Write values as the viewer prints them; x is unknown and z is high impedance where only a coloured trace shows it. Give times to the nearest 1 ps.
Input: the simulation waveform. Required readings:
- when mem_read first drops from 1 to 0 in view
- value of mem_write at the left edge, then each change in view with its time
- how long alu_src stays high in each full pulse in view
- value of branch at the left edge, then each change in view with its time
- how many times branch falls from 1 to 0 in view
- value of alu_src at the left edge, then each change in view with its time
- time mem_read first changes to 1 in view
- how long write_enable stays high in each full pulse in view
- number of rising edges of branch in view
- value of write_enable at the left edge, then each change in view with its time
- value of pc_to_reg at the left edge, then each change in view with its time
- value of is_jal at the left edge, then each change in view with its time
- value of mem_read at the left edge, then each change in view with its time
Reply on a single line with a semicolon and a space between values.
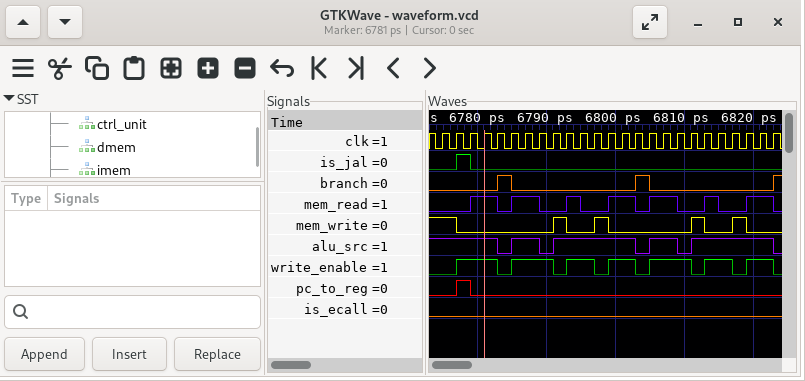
6783 ps; 1, 0 at 6777 ps, 1 at 6791 ps, 0 at 6793 ps, 1 at 6797 ps, 0 at 6799 ps, 1 at 6811 ps, 0 at 6813 ps, 1 at 6817 ps, 0 at 6819 ps; 4 ps, 12 ps, 4 ps, 12 ps; 0, 1 at 6783 ps, 0 at 6785 ps, 1 at 6803 ps, 0 at 6805 ps, 1 at 6823 ps; 2; 1, 0 at 6783 ps, 1 at 6785 ps, 0 at 6789 ps, 1 at 6791 ps, 0 at 6803 ps, 1 at 6805 ps, 0 at 6809 ps, 1 at 6811 ps, 0 at 6823 ps; 6779 ps; 6 ps, 6 ps, 4 ps, 4 ps, 6 ps, 4 ps, 4 ps; 3; 0, 1 at 6777 ps, 0 at 6783 ps, 1 at 6785 ps, 0 at 6791 ps, 1 at 6793 ps, 0 at 6797 ps, 1 at 6799 ps, 0 at 6803 ps, 1 at 6805 ps, 0 at 6811 ps, 1 at 6813 ps, 0 at 6817 ps, 1 at 6819 ps, 0 at 6823 ps; 0, 1 at 6777 ps, 0 at 6779 ps; 0, 1 at 6777 ps, 0 at 6779 ps; 0, 1 at 6779 ps, 0 at 6783 ps, 1 at 6785 ps, 0 at 6789 ps, 1 at 6793 ps, 0 at 6795 ps, 1 at 6799 ps, 0 at 6803 ps, 1 at 6805 ps, 0 at 6809 ps, 1 at 6813 ps, 0 at 6815 ps, 1 at 6819 ps, 0 at 6823 ps
